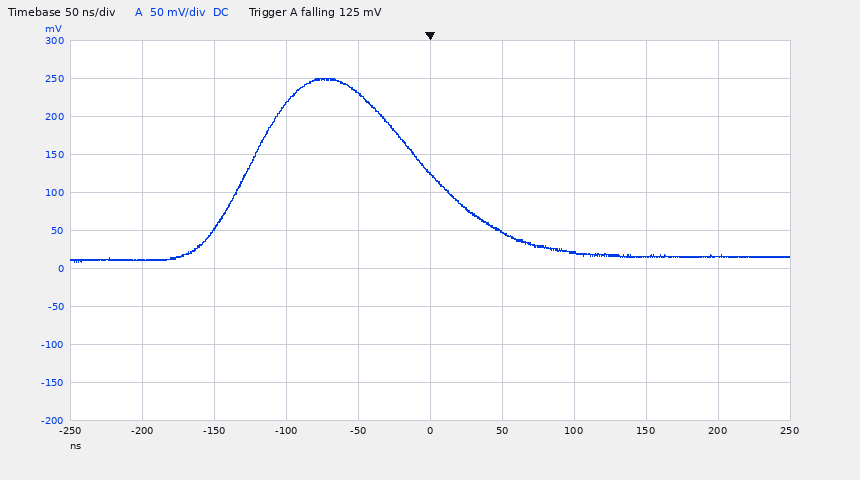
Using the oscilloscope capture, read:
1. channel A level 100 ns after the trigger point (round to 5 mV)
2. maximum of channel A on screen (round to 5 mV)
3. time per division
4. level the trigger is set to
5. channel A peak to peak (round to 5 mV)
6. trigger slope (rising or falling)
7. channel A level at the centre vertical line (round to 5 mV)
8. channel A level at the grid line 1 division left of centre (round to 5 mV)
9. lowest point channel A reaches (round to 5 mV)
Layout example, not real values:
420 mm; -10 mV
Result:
20 mV; 250 mV; 50 ns; 125 mV; 240 mV; falling; 125 mV; 230 mV; 10 mV
